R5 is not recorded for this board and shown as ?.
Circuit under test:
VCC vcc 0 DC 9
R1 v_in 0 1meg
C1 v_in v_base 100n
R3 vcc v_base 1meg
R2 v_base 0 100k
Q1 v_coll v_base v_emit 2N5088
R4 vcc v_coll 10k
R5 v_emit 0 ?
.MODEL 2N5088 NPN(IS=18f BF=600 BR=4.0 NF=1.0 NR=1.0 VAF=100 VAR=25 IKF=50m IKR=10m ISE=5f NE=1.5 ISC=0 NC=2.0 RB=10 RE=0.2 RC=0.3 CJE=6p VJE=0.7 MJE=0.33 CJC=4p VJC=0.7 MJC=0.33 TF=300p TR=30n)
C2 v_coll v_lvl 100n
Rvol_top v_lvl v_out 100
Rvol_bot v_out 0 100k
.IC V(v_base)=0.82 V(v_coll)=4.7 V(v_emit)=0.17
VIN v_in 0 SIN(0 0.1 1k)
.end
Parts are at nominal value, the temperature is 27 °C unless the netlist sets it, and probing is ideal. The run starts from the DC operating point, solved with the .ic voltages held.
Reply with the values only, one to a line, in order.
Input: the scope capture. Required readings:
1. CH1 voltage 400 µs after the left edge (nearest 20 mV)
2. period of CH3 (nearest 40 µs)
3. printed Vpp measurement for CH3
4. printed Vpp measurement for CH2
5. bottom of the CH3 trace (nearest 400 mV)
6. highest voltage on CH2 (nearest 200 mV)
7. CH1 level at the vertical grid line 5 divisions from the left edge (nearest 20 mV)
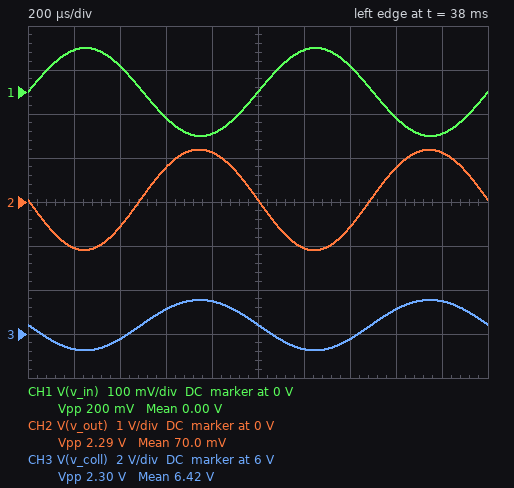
60 mV
1.00 ms
2.30 V
2.29 V
5.2 V
1.2 V
0 V
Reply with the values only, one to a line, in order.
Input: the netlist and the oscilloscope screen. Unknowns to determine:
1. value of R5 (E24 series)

680 Ω
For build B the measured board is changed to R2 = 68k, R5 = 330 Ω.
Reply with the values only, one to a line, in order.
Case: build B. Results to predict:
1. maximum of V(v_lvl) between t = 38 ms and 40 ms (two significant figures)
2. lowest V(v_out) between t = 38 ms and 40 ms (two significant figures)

830 mV
-1.0 V
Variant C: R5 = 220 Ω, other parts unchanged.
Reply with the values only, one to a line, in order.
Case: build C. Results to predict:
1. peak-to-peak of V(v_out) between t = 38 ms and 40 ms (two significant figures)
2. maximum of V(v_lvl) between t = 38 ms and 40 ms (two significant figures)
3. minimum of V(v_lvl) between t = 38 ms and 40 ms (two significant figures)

6.4 V
3.1 V
-3.4 V
